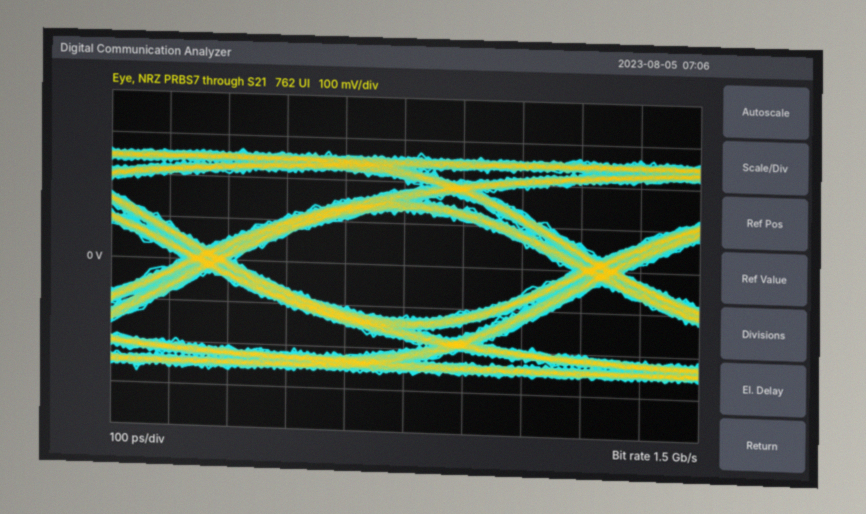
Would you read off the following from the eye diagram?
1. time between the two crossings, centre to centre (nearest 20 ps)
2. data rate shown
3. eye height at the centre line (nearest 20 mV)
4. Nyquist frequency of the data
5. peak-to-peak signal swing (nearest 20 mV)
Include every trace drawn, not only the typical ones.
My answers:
660 ps
1.5 Gb/s
260 mV
750 MHz
540 mV
